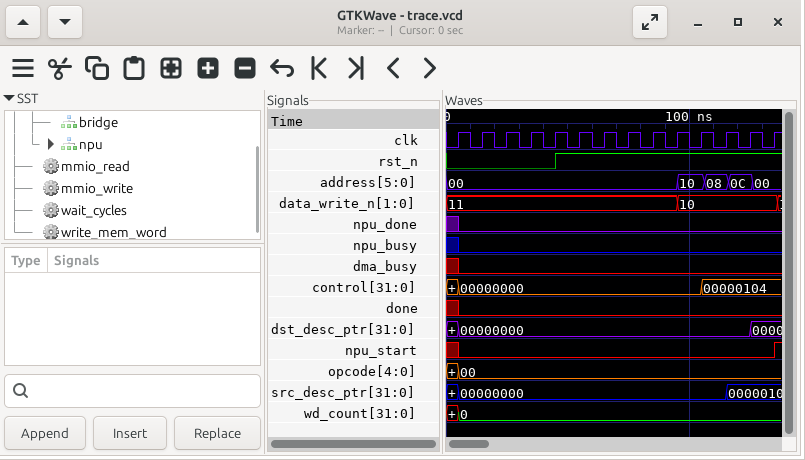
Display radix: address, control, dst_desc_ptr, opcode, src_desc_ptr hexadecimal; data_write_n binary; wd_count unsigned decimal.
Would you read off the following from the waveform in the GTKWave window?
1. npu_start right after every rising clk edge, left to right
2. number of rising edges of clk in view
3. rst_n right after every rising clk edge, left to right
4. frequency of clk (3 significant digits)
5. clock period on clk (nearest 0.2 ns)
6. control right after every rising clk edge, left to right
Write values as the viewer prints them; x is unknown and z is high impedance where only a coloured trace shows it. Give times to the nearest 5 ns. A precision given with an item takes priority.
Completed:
0 0 0 0 0 0 0 0 0 0 0 0 0 1
14
0 0 0 0 1 1 1 1 1 1 1 1 1 1
100 MHz
10 ns
00000000, 00000000, 00000000, 00000000, 00000000, 00000000, 00000000, 00000000, 00000000, 00000000, 00000104, 00000104, 00000104, 00000104
